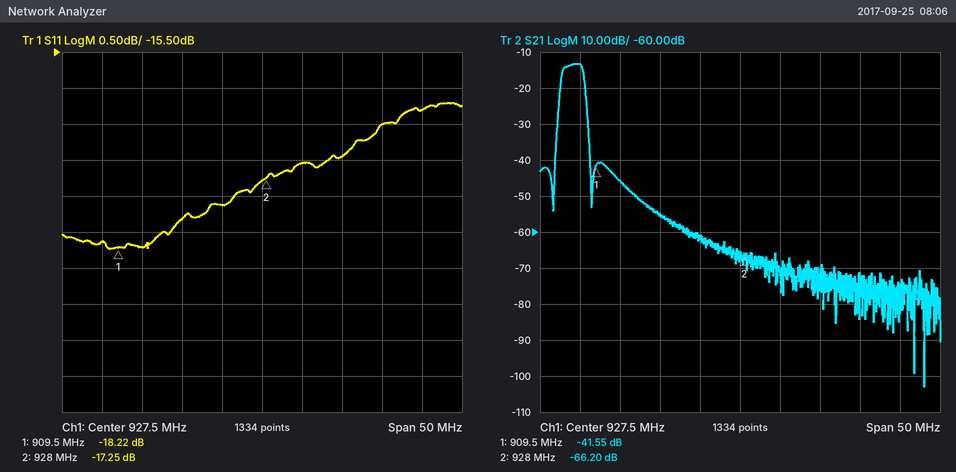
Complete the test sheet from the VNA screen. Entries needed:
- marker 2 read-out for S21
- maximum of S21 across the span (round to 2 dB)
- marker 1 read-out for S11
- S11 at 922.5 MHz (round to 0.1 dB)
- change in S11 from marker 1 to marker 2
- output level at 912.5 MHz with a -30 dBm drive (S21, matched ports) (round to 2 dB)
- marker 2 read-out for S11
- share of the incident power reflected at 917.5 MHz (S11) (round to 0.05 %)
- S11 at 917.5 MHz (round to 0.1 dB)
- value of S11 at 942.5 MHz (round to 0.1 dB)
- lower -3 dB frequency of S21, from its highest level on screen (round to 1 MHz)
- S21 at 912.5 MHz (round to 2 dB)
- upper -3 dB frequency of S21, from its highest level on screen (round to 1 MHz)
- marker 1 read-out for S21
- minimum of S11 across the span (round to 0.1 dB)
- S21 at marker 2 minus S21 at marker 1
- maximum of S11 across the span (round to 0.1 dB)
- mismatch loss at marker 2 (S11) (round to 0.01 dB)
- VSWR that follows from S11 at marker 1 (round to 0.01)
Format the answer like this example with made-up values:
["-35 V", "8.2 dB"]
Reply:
["-66.20 dB", "-14 dB", "-18.22 dB", "-17.6 dB", "0.97 dB", "-76 dBm", "-17.25 dB", "1.65 %", "-17.8 dB", "-16.5 dB", "905 MHz", "-46 dB", "908 MHz", "-41.55 dB", "-18.2 dB", "-24.65 dB", "-16.2 dB", "0.08 dB", "1.28"]
